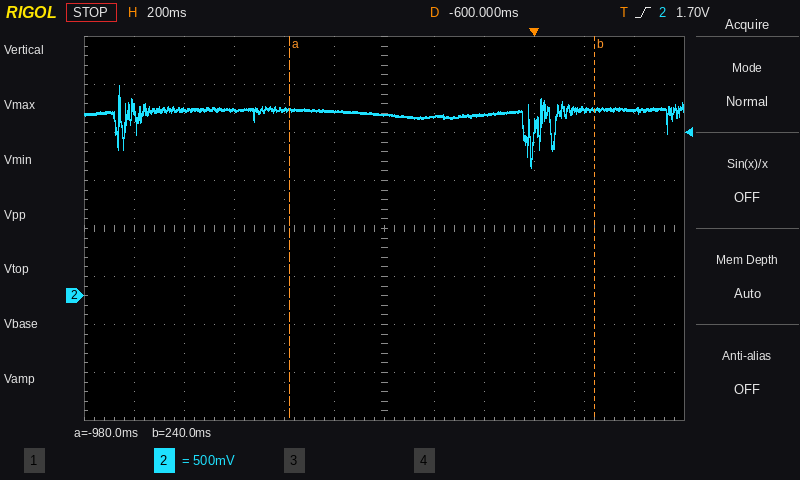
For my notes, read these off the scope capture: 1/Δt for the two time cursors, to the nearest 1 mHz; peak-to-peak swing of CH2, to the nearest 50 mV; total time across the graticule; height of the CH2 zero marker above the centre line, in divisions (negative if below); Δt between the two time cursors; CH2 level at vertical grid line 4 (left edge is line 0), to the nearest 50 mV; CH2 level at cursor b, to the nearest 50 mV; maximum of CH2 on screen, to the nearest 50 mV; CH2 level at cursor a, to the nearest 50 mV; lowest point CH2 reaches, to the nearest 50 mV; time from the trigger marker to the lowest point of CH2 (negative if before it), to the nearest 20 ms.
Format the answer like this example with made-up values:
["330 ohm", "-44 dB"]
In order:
["820 mHz", "850 mV", "2.4 s", "-1.4 div", "1.22 s", "1.95 V", "1.95 V", "2.20 V", "1.95 V", "1.35 V", "-20 ms"]
